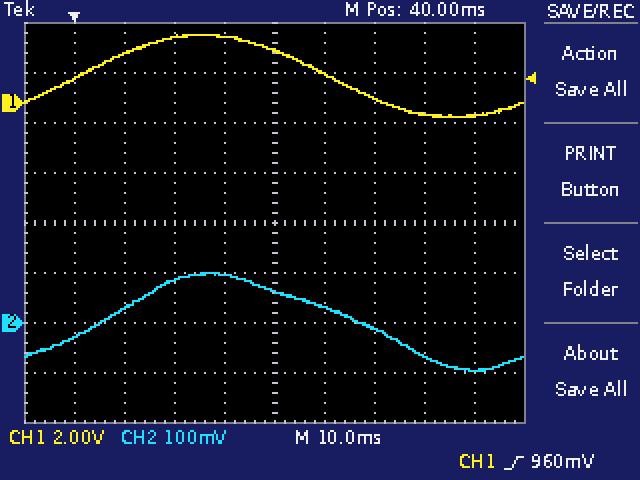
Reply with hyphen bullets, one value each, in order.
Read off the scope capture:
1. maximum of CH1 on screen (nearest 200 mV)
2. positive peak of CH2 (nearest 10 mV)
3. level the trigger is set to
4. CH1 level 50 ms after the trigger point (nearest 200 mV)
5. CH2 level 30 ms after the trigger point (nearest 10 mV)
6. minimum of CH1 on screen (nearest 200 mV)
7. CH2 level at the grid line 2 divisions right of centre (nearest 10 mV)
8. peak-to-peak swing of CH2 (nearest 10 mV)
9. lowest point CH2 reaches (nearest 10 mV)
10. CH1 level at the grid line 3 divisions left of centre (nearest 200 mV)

- 2.8 V
- 100 mV
- 960 mV
- 1.2 V
- 100 mV
- -600 mV
- -10 mV
- 200 mV
- -100 mV
- 2.0 V
